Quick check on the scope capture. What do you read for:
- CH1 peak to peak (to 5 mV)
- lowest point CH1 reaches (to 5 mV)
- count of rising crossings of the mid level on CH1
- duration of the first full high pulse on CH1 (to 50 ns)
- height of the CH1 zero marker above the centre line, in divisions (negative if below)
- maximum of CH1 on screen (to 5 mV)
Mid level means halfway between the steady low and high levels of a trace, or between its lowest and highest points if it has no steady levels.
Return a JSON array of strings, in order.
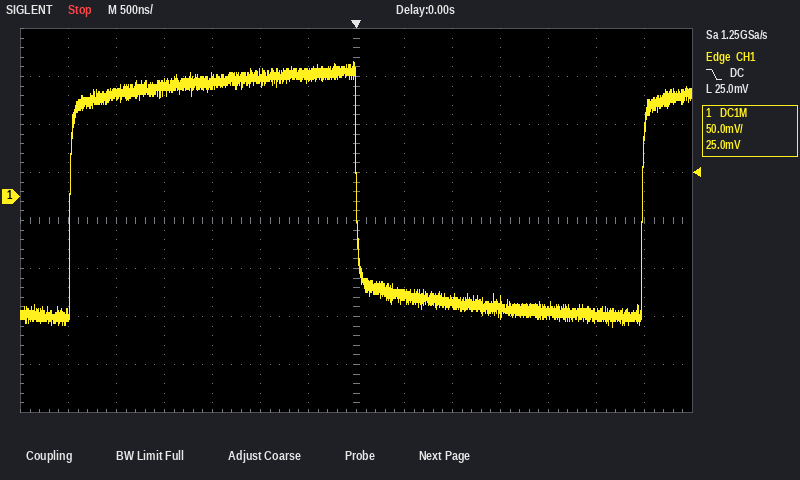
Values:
["275 mV", "-135 mV", "2", "3.00 µs", "+0.5 div", "140 mV"]
